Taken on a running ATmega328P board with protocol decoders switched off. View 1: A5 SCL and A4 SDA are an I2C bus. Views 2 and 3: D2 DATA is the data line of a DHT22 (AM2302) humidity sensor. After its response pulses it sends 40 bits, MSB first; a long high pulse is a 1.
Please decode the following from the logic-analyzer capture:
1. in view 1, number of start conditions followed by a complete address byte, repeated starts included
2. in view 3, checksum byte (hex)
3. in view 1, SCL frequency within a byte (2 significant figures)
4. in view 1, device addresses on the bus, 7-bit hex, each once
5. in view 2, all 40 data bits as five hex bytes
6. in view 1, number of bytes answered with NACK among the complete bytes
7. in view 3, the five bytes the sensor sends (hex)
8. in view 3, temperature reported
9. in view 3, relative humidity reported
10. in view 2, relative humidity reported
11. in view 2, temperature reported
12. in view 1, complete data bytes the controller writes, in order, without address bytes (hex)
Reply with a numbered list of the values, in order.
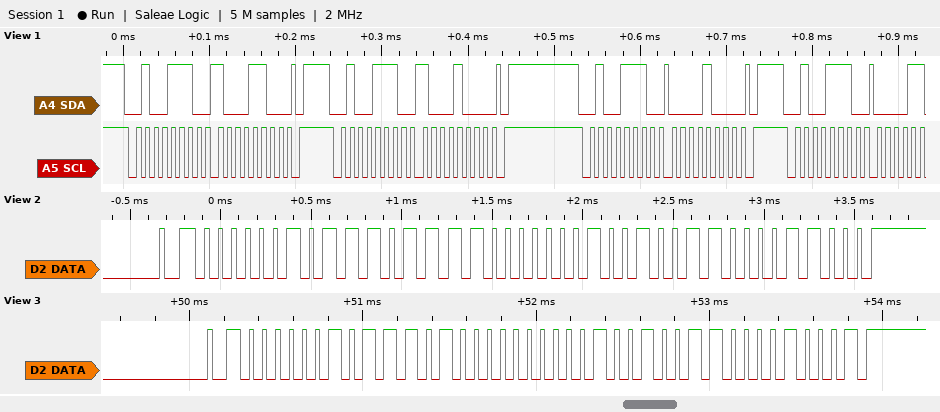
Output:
1. 4
2. 0x11
3. 100 kHz
4. 0x27
5. 02 EF 01 26 18
6. 0
7. 02 E8 01 26 11
8. 29.4 °C
9. 74.4 %
10. 75.1 %
11. 29.4 °C
12. 8C 88 08
